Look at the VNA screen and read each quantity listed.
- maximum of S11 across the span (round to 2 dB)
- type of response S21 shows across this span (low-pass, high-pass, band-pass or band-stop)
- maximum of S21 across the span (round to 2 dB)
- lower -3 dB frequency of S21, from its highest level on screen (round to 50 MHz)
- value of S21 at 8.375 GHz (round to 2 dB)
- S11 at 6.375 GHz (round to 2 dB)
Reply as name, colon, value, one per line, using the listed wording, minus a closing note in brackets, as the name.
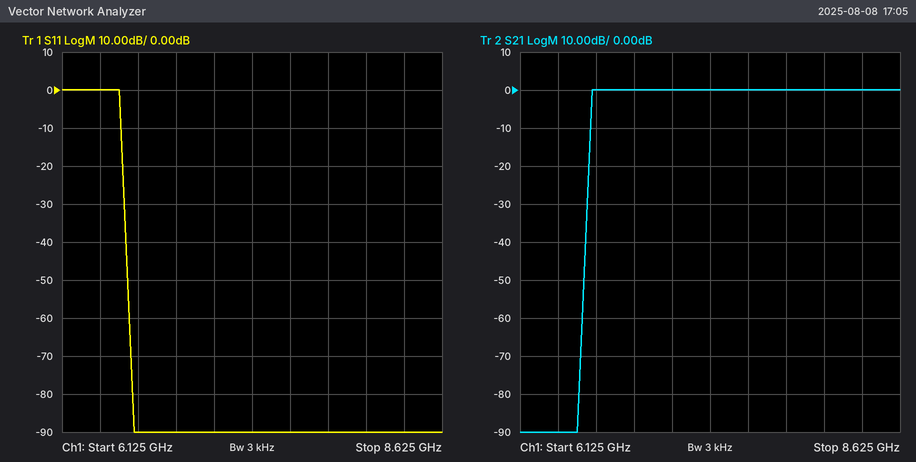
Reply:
maximum of S11 across the span: 0 dB
type of response S21 shows across this span: high-pass
maximum of S21 across the span: 0 dB
lower -3 dB frequency of S21, from its highest level on screen: 6.60 GHz
value of S21 at 8.375 GHz: 0 dB
S11 at 6.375 GHz: 0 dB
